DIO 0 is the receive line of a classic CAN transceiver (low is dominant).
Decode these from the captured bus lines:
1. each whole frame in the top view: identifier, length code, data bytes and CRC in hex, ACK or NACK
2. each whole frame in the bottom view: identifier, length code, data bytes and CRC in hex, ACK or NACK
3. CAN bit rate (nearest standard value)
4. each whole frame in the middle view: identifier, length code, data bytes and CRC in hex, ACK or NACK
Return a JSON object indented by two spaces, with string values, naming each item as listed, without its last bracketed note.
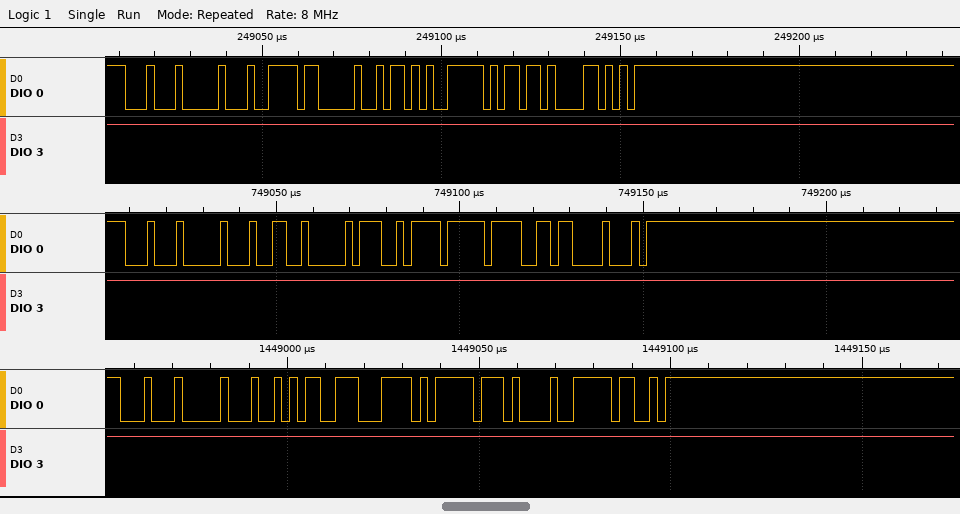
{
  "each whole frame in the top view: identifier, length code, data bytes and CRC in hex, ACK or NACK": "ID 110, DLC 4, data F6 02 D4 FD, CRC 5A1A, ACK",
  "each whole frame in the bottom view: identifier, length code, data bytes and CRC in hex, ACK or NACK": "ID 110, DLC 4, data AC E3 D7 FA, CRC 09FC, ACK",
  "CAN bit rate": "500 kbit/s",
  "each whole frame in the middle view: identifier, length code, data bytes and CRC in hex, ACK or NACK": "ID 110, DLC 4, data C8 1C BD FF, CRC 1B08, ACK"
}
